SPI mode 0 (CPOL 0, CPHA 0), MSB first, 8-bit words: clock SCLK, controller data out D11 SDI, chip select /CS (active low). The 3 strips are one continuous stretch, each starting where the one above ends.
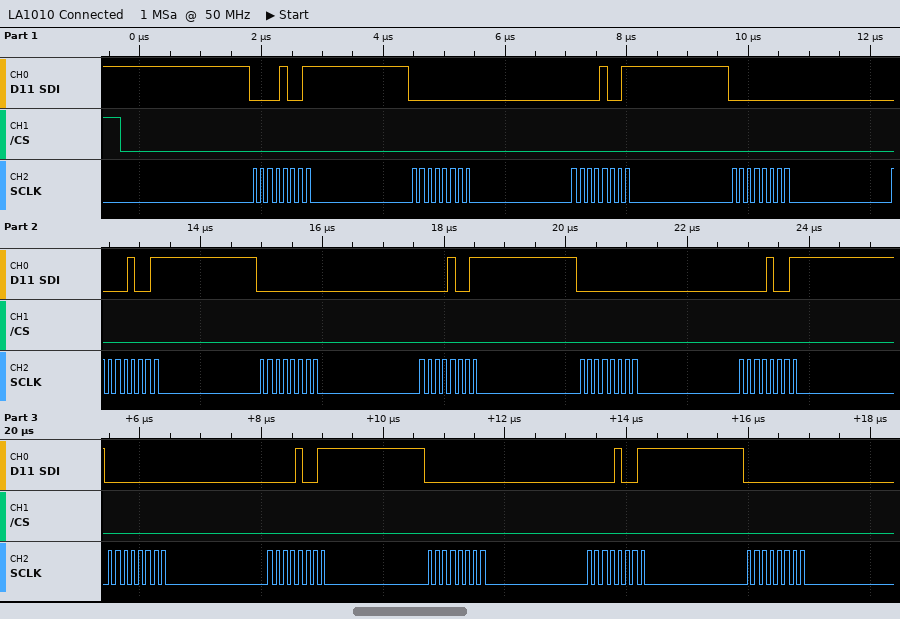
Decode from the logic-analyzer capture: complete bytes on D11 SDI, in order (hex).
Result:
09 00 09 00 09 00 09 00 09 00 09 00 09 00
